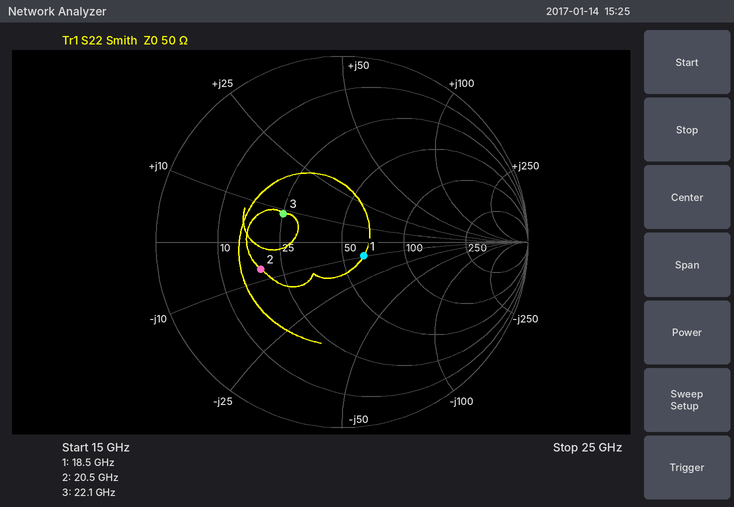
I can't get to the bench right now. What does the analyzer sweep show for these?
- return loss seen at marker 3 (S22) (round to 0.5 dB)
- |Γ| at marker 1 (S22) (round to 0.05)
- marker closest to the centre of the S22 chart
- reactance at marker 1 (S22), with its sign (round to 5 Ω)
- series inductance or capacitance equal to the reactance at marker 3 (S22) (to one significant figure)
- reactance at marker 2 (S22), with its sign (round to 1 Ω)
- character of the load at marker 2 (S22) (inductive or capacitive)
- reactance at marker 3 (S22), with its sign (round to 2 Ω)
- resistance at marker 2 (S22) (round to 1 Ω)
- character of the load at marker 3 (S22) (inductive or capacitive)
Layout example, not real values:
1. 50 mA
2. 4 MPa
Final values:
1. 9.0 dB
2. 0.15
3. marker 1
4. -10 Ω
5. 60 pH
6. -7 Ω
7. capacitive
8. +8 Ω
9. 19 Ω
10. inductive
